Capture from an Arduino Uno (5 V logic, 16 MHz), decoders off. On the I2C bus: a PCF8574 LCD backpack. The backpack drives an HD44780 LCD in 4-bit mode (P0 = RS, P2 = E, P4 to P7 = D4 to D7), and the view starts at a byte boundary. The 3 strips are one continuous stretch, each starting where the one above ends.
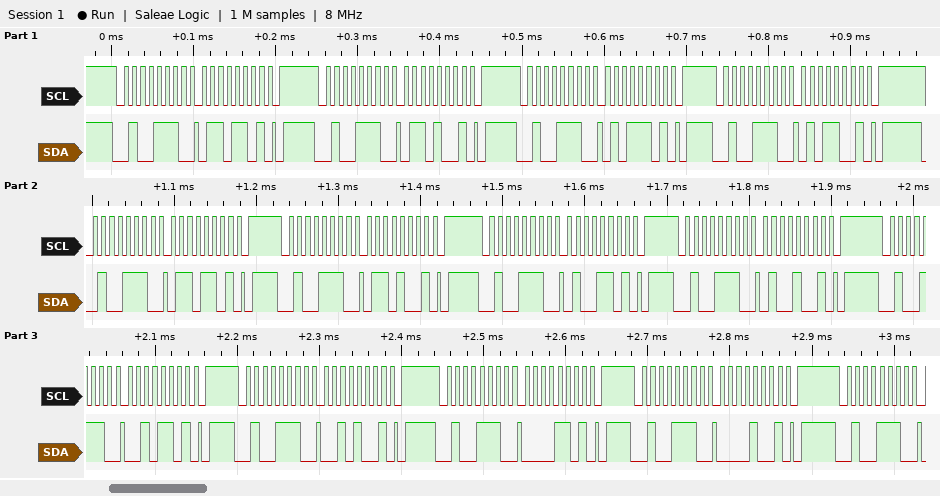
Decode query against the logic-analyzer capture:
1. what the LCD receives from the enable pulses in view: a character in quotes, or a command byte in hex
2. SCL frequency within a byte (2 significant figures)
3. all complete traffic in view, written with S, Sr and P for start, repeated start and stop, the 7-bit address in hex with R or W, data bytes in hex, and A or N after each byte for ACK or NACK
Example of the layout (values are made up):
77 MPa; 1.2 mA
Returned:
'e' 'd' ' '; 100 kHz; S 27W A 6D A P S 27W A 69 A P S 27W A 5D A P S 27W A 59 A P S 27W A 6D A P S 27W A 69 A P S 27W A 4D A P S 27W A 49 A P S 27W A 2D A P S 27W A 29 A P S 27W A 0D A P S 27W A 09 A P S 27W A
